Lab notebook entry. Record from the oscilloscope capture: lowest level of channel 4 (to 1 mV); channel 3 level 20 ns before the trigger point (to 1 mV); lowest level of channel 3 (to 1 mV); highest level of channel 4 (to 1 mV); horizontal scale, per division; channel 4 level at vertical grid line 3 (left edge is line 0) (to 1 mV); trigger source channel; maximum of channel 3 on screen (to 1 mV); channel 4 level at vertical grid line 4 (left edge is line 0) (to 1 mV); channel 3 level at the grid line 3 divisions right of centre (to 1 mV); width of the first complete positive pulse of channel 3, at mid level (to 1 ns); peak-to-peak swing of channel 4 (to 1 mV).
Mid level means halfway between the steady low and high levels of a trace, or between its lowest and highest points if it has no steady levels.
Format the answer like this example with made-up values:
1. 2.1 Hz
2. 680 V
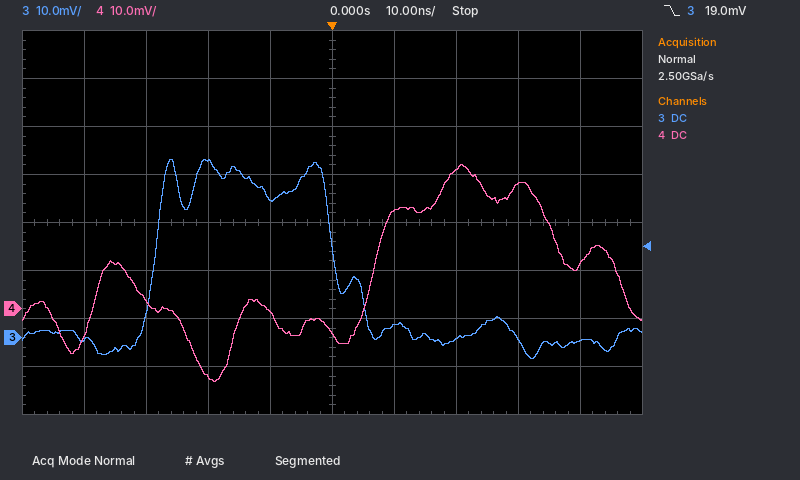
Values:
1. -15 mV
2. 37 mV
3. -4 mV
4. 30 mV
5. 10 ns
6. -14 mV
7. channel 3
8. 37 mV
9. -1 mV
10. 0 mV
11. 29 ns
12. 45 mV
